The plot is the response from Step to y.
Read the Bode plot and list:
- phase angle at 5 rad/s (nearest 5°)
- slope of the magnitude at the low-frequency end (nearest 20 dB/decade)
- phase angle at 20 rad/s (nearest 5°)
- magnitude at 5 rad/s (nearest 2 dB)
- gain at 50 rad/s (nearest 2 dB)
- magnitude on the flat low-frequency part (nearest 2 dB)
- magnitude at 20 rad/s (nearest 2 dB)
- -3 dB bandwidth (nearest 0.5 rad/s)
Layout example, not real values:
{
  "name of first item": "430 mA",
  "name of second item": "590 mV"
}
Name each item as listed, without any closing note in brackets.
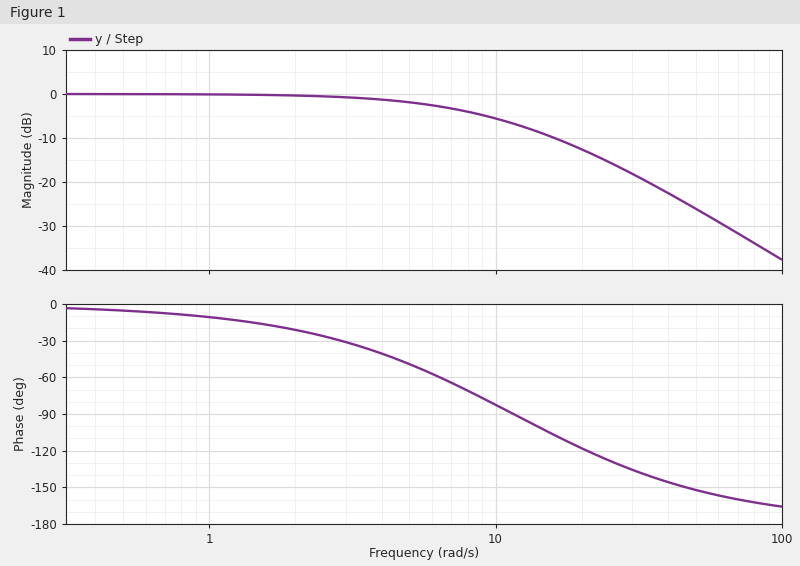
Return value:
{
  "phase angle at 5 rad/s": "-50°",
  "slope of the magnitude at the low-frequency end": "0 dB/decade",
  "phase angle at 20 rad/s": "-120°",
  "magnitude at 5 rad/s": "-2 dB",
  "gain at 50 rad/s": "-26 dB",
  "magnitude on the flat low-frequency part": "0 dB",
  "magnitude at 20 rad/s": "-12 dB",
  "-3 dB bandwidth": "6.5 rad/s"
}
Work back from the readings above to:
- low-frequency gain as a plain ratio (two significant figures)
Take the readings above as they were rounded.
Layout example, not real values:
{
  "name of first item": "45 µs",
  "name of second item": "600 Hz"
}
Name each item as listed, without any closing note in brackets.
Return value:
{
  "low-frequency gain as a plain ratio": "1.0"
}
